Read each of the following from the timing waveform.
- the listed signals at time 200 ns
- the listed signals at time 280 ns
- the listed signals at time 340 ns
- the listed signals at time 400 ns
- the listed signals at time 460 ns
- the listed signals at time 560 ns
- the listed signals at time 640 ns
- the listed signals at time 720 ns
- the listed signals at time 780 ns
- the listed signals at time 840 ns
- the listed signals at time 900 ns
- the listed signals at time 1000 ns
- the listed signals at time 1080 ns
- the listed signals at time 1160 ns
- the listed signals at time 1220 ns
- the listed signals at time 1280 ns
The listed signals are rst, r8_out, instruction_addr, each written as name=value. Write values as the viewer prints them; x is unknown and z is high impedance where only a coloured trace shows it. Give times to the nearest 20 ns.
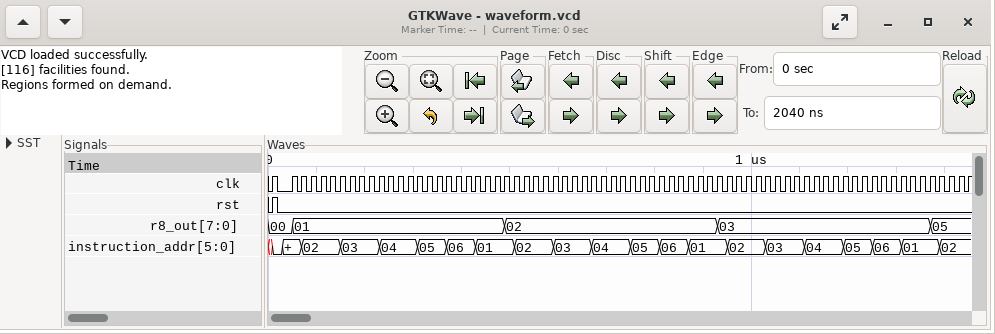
rst=0, r8_out=01, instruction_addr=03
rst=0, r8_out=01, instruction_addr=04
rst=0, r8_out=01, instruction_addr=05
rst=0, r8_out=01, instruction_addr=06
rst=0, r8_out=01, instruction_addr=01
rst=0, r8_out=02, instruction_addr=02
rst=0, r8_out=02, instruction_addr=03
rst=0, r8_out=02, instruction_addr=04
rst=0, r8_out=02, instruction_addr=05
rst=0, r8_out=02, instruction_addr=06
rst=0, r8_out=02, instruction_addr=01
rst=0, r8_out=03, instruction_addr=02
rst=0, r8_out=03, instruction_addr=03
rst=0, r8_out=03, instruction_addr=04
rst=0, r8_out=03, instruction_addr=05
rst=0, r8_out=03, instruction_addr=06
